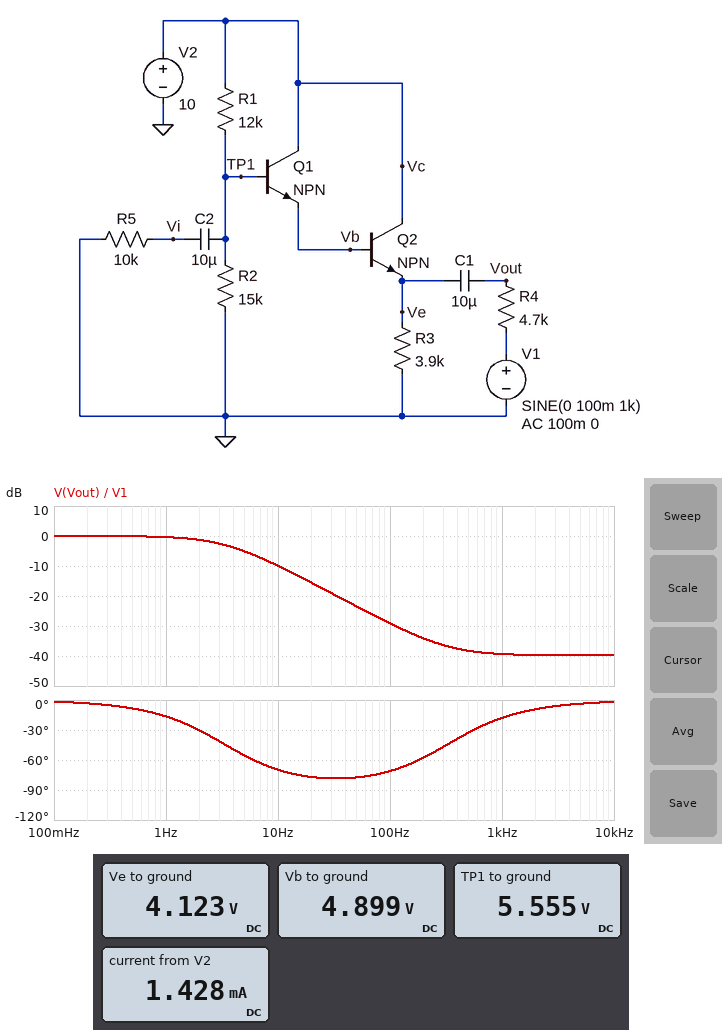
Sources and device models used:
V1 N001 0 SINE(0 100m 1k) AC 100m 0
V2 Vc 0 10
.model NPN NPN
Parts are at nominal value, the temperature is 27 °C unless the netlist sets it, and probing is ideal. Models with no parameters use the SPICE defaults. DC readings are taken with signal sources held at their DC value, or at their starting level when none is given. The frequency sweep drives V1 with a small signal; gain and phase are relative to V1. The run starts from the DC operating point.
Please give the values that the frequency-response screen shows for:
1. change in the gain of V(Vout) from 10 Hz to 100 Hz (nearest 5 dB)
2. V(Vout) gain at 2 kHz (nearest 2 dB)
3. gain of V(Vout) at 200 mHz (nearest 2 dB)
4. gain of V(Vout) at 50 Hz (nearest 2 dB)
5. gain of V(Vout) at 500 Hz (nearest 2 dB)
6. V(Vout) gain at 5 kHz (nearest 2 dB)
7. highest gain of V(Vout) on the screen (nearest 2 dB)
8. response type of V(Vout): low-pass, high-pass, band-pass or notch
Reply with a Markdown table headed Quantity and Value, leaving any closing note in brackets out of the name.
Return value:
| Quantity | Value |
|---|---|
| change in the gain of V(Vout) from 10 Hz to 100 Hz | -20 dB |
| V(Vout) gain at 2 kHz | -40 dB |
| gain of V(Vout) at 200 mHz | 0 dB |
| gain of V(Vout) at 50 Hz | -24 dB |
| gain of V(Vout) at 500 Hz | -38 dB |
| V(Vout) gain at 5 kHz | -40 dB |
| highest gain of V(Vout) on the screen | 0 dB |
| response type of V(Vout): low-pass, high-pass, band-pass or notch | low-pass |
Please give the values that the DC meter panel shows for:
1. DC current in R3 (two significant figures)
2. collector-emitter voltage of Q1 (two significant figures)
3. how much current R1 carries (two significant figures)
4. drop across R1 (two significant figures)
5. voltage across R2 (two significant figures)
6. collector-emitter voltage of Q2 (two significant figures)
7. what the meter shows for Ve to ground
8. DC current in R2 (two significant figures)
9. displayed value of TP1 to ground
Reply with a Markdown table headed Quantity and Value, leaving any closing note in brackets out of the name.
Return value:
| Quantity | Value |
|---|---|
| DC current in R3 | 1.1 mA |
| collector-emitter voltage of Q1 | 5.1 V |
| how much current R1 carries | 370 µA |
| drop across R1 | 4.4 V |
| voltage across R2 | 5.6 V |
| collector-emitter voltage of Q2 | 5.9 V |
| what the meter shows for Ve to ground | 4.123 V |
| DC current in R2 | 370 µA |
| displayed value of TP1 to ground | 5.555 V |
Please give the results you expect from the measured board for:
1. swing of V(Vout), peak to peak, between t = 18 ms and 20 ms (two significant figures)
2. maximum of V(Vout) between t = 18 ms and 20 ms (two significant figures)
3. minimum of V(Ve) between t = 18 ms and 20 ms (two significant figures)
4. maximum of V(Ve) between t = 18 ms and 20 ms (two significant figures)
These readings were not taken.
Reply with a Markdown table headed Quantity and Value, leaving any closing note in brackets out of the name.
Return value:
| Quantity | Value |
|---|---|
| swing of V(Vout), peak to peak, between t = 18 ms and 20 ms | 2.2 mV |
| maximum of V(Vout) between t = 18 ms and 20 ms | 1.3 mV |
| minimum of V(Ve) between t = 18 ms and 20 ms | 4.1 V |
| maximum of V(Ve) between t = 18 ms and 20 ms | 4.1 V |
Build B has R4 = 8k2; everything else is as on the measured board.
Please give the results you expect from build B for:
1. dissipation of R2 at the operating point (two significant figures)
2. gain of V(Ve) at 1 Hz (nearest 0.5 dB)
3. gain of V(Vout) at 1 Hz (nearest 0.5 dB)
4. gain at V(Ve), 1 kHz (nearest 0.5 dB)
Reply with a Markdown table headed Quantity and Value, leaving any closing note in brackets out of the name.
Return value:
| Quantity | Value |
|---|---|
| dissipation of R2 at the operating point | 2.1 mW |
| gain of V(Ve) at 1 Hz | -51.5 dB |
| gain of V(Vout) at 1 Hz | -1.0 dB |
| gain at V(Ve), 1 kHz | -44.5 dB |
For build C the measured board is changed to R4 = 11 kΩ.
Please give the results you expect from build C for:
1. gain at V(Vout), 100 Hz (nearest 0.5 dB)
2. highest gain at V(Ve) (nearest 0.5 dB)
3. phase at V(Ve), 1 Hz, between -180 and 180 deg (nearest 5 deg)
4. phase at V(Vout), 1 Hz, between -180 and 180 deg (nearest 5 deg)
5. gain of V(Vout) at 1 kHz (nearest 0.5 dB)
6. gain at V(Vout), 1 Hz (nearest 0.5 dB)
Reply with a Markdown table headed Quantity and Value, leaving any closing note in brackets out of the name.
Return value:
| Quantity | Value |
|---|---|
| gain at V(Vout), 100 Hz | -36.5 dB |
| highest gain at V(Ve) | -47.0 dB |
| phase at V(Ve), 1 Hz, between -180 and 180 deg | 55 deg |
| phase at V(Vout), 1 Hz, between -180 and 180 deg | -35 deg |
| gain of V(Vout) at 1 kHz | -46.5 dB |
| gain at V(Vout), 1 Hz | -1.5 dB |
